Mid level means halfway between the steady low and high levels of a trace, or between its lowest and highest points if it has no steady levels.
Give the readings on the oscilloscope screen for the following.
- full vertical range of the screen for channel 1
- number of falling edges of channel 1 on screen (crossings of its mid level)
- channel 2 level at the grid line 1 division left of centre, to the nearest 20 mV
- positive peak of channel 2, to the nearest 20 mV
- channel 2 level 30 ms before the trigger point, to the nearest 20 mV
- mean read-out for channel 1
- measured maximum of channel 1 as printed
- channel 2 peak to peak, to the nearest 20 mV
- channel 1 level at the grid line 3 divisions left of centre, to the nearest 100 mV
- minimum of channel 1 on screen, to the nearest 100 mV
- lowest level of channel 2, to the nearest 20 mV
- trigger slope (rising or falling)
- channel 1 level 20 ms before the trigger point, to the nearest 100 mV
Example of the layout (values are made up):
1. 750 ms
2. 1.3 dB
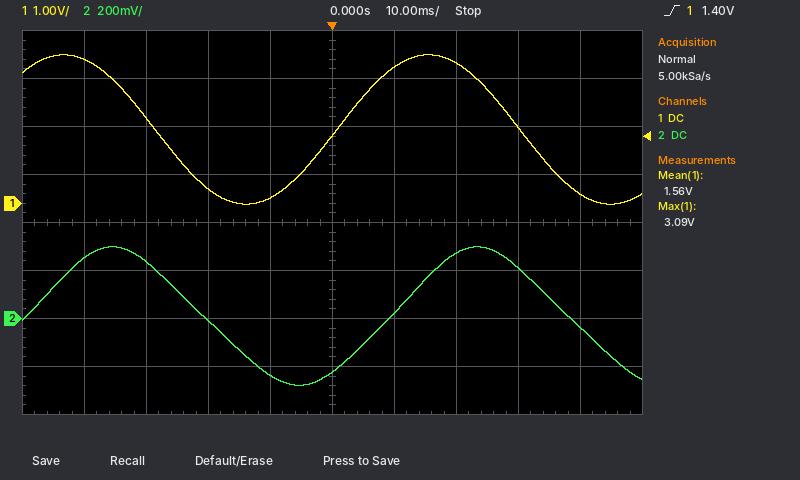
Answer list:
1. 8 V
2. 2
3. -240 mV
4. 300 mV
5. 240 mV
6. 1.56 V
7. 3.09 V
8. 580 mV
9. 1.8 V
10. 0.0 V
11. -280 mV
12. rising
13. 300 mV
